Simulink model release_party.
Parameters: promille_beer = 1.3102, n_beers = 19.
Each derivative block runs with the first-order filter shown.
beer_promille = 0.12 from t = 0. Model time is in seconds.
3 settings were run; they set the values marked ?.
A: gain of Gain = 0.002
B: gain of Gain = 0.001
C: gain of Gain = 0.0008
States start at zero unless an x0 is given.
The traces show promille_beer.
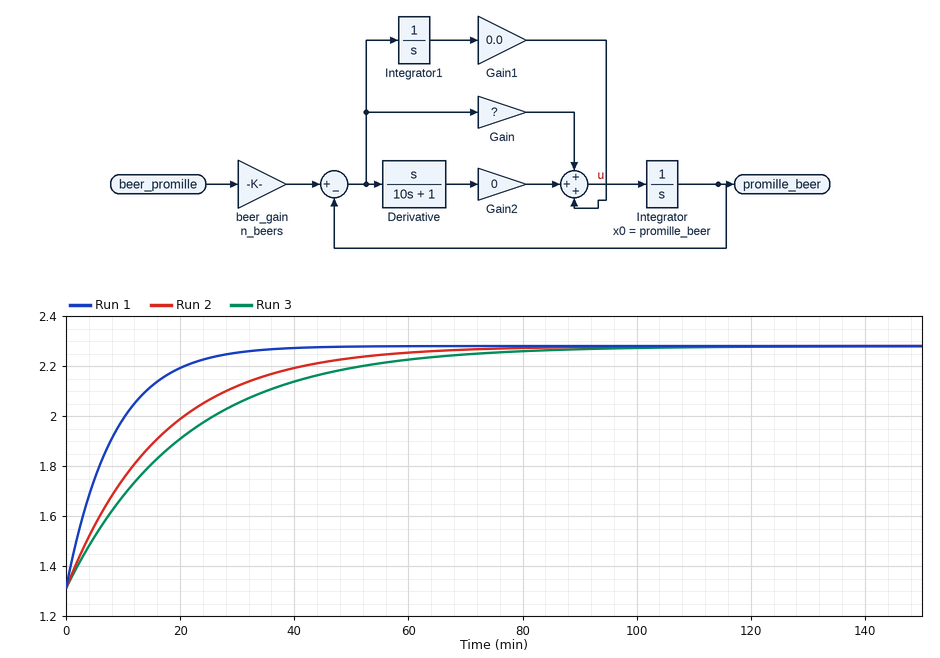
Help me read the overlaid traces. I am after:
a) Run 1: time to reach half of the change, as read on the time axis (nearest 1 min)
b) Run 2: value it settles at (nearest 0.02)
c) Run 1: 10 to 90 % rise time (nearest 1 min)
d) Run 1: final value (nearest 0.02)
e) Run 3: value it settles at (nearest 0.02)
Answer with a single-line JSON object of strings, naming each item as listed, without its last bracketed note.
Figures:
{"Run 1: time to reach half of the change, as read on the time axis": "6 min", "Run 2: value it settles at": "2.28", "Run 1: 10 to 90 % rise time": "18 min", "Run 1: final value": "2.28", "Run 3: value it settles at": "2.28"}
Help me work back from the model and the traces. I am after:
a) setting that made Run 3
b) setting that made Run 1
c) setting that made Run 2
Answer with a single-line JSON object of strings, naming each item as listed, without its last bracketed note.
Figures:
{"setting that made Run 3": "C", "setting that made Run 1": "A", "setting that made Run 2": "B"}
